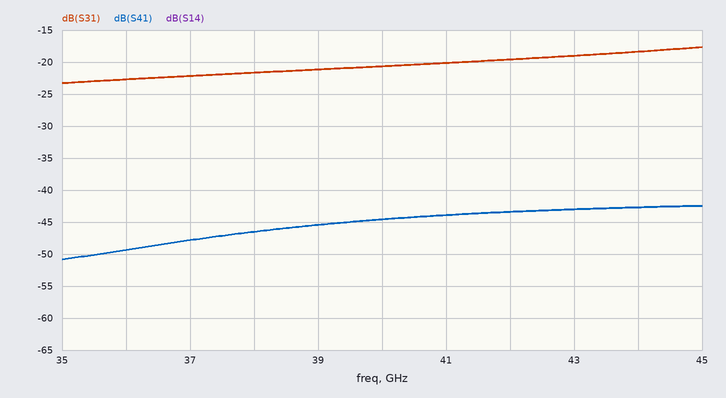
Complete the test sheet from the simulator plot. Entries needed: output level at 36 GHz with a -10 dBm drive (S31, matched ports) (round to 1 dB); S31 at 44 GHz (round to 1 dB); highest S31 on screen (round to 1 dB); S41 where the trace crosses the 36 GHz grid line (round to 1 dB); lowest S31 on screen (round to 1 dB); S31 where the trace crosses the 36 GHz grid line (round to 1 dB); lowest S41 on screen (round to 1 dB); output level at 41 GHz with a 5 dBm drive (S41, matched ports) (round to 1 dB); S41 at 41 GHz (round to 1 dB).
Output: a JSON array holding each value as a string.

["-33 dBm", "-18 dB", "-18 dB", "-49 dB", "-23 dB", "-23 dB", "-51 dB", "-39 dBm", "-44 dB"]
